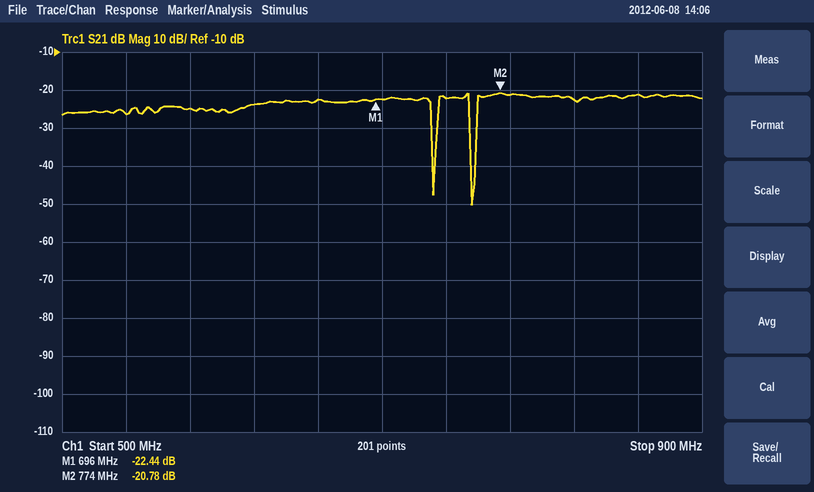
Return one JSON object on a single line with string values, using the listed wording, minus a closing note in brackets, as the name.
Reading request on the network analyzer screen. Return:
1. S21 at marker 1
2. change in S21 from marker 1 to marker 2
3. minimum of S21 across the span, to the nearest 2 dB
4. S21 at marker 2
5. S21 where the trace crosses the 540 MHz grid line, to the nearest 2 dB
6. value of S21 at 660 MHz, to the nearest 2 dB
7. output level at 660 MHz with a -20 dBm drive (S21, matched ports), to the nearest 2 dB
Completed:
{"S21 at marker 1": "-22.44 dB", "change in S21 from marker 1 to marker 2": "1.66 dB", "minimum of S21 across the span, to the nearest 2 dB": "-50 dB", "S21 at marker 2": "-20.78 dB", "S21 where the trace crosses the 540 MHz grid line, to the nearest 2 dB": "-26 dB", "value of S21 at 660 MHz, to the nearest 2 dB": "-22 dB", "output level at 660 MHz with a -20 dBm drive (S21, matched ports), to the nearest 2 dB": "-42 dBm"}
